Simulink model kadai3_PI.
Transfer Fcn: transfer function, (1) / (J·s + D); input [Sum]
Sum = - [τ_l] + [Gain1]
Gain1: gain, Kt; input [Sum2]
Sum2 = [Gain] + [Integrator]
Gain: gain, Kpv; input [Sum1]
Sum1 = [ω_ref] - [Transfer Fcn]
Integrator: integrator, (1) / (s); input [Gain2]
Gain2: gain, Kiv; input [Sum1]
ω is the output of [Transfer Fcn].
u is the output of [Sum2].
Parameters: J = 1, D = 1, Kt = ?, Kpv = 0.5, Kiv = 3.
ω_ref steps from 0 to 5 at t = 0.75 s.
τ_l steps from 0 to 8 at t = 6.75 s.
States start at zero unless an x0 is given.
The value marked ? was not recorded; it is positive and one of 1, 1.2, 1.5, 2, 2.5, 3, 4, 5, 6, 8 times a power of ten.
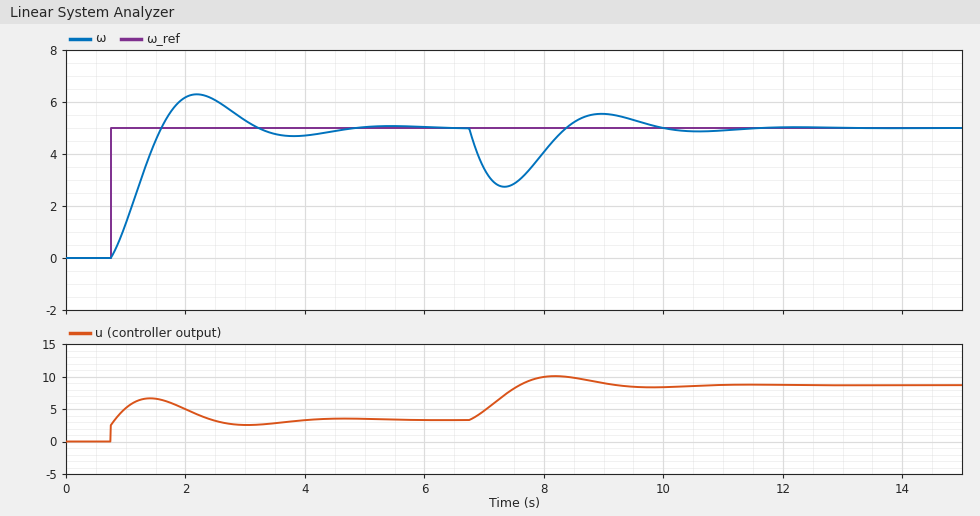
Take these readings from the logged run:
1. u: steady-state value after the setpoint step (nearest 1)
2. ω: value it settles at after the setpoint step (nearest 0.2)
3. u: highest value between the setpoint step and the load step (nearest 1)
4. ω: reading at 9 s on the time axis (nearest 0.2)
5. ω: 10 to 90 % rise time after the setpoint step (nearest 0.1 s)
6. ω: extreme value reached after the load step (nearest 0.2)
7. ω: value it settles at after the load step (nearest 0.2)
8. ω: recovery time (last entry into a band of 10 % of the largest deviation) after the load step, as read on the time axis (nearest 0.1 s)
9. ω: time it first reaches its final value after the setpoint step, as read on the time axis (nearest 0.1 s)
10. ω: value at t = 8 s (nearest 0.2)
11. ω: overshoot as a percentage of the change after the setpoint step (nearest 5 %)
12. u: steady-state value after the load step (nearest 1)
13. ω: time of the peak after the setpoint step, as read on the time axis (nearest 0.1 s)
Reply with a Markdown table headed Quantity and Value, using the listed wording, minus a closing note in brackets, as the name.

| Quantity | Value |
|---|---|
| u: steady-state value after the setpoint step | 3 |
| ω: value it settles at after the setpoint step | 5.0 |
| u: highest value between the setpoint step and the load step | 7 |
| ω: reading at 9 s on the time axis | 5.6 |
| ω: 10 to 90 % rise time after the setpoint step | 0.6 s |
| ω: extreme value reached after the load step | 2.8 |
| ω: value it settles at after the load step | 5.0 |
| ω: recovery time (last entry into a band of 10 % of the largest deviation) after the load step, as read on the time axis | 9.6 s |
| ω: time it first reaches its final value after the setpoint step, as read on the time axis | 1.6 s |
| ω: value at t = 8 s | 4.0 |
| ω: overshoot as a percentage of the change after the setpoint step | 25 % |
| u: steady-state value after the load step | 9 |
| ω: time of the peak after the setpoint step, as read on the time axis | 2.2 s |
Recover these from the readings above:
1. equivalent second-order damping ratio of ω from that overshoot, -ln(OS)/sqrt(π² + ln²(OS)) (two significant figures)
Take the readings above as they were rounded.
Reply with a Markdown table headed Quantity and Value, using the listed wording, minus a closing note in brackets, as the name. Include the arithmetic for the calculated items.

| Quantity | Value |
|---|---|
| equivalent second-order damping ratio of ω from that overshoot, -ln(OS)/sqrt(π² + ln²(OS)) | ln(0.25) = -1.386; 1.386 / sqrt(9.870 + 1.922) = 0.40 |
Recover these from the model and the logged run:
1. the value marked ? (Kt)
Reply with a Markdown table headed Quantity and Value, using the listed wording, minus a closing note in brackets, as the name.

| Quantity | Value |
|---|---|
| the value marked ? | 1.5 |
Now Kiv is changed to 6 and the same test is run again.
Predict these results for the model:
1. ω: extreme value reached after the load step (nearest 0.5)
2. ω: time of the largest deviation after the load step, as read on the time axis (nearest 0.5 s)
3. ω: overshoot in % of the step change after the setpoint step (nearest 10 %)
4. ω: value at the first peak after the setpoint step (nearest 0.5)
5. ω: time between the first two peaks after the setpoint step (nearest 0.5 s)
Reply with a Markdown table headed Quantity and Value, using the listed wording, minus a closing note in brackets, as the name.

| Quantity | Value |
|---|---|
| ω: extreme value reached after the load step | 3.0 |
| ω: time of the largest deviation after the load step, as read on the time axis | 7.0 s |
| ω: overshoot in % of the step change after the setpoint step | 40 % |
| ω: value at the first peak after the setpoint step | 7.0 |
| ω: time between the first two peaks after the setpoint step | 2.0 s |
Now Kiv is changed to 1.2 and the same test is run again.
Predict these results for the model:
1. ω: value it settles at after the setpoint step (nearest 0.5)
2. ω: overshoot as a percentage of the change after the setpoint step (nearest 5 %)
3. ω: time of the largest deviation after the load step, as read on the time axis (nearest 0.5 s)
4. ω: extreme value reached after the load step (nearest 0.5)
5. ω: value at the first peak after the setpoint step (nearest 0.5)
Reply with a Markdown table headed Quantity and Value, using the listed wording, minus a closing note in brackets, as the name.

| Quantity | Value |
|---|---|
| ω: value it settles at after the setpoint step | 5.0 |
| ω: overshoot as a percentage of the change after the setpoint step | 10 % |
| ω: time of the largest deviation after the load step, as read on the time axis | 7.5 s |
| ω: extreme value reached after the load step | 2.0 |
| ω: value at the first peak after the setpoint step | 5.5 |
